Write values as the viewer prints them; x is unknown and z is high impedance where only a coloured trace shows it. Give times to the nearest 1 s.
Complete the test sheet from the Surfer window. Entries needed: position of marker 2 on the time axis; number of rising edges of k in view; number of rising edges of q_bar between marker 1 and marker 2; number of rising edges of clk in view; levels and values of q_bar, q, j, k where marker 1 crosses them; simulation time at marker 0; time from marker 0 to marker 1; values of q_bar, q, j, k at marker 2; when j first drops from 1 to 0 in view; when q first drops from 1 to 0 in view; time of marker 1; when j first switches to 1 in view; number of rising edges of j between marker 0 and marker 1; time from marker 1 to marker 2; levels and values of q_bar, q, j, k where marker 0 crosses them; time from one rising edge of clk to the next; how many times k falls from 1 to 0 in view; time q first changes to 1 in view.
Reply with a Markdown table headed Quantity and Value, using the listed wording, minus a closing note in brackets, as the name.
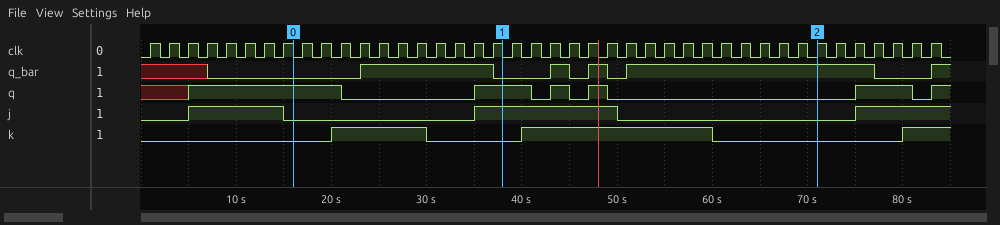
| Quantity | Value |
|---|---|
| position of marker 2 on the time axis | 71 s |
| number of rising edges of k in view | 3 |
| number of rising edges of q_bar between marker 1 and marker 2 | 3 |
| number of rising edges of clk in view | 42 |
| levels and values of q_bar, q, j, k where marker 1 crosses them | q_bar=0, q=1, j=1, k=0 |
| simulation time at marker 0 | 16 s |
| time from marker 0 to marker 1 | 22 s |
| values of q_bar, q, j, k at marker 2 | q_bar=1, q=0, j=0, k=0 |
| when j first drops from 1 to 0 in view | 15 s |
| when q first drops from 1 to 0 in view | 21 s |
| time of marker 1 | 38 s |
| when j first switches to 1 in view | 5 s |
| number of rising edges of j between marker 0 and marker 1 | 1 |
| time from marker 1 to marker 2 | 33 s |
| levels and values of q_bar, q, j, k where marker 0 crosses them | q_bar=0, q=1, j=0, k=0 |
| time from one rising edge of clk to the next | 2 s |
| how many times k falls from 1 to 0 in view | 2 |
| time q first changes to 1 in view | 5 s |
